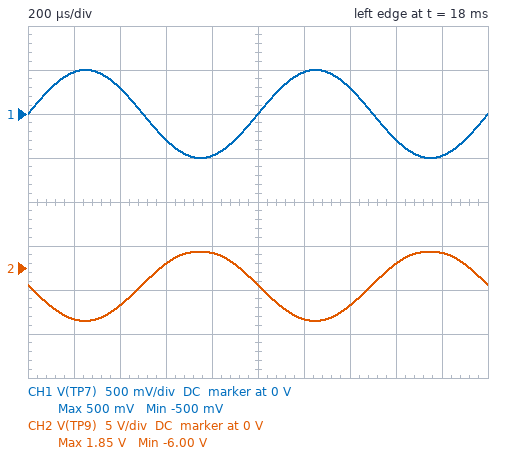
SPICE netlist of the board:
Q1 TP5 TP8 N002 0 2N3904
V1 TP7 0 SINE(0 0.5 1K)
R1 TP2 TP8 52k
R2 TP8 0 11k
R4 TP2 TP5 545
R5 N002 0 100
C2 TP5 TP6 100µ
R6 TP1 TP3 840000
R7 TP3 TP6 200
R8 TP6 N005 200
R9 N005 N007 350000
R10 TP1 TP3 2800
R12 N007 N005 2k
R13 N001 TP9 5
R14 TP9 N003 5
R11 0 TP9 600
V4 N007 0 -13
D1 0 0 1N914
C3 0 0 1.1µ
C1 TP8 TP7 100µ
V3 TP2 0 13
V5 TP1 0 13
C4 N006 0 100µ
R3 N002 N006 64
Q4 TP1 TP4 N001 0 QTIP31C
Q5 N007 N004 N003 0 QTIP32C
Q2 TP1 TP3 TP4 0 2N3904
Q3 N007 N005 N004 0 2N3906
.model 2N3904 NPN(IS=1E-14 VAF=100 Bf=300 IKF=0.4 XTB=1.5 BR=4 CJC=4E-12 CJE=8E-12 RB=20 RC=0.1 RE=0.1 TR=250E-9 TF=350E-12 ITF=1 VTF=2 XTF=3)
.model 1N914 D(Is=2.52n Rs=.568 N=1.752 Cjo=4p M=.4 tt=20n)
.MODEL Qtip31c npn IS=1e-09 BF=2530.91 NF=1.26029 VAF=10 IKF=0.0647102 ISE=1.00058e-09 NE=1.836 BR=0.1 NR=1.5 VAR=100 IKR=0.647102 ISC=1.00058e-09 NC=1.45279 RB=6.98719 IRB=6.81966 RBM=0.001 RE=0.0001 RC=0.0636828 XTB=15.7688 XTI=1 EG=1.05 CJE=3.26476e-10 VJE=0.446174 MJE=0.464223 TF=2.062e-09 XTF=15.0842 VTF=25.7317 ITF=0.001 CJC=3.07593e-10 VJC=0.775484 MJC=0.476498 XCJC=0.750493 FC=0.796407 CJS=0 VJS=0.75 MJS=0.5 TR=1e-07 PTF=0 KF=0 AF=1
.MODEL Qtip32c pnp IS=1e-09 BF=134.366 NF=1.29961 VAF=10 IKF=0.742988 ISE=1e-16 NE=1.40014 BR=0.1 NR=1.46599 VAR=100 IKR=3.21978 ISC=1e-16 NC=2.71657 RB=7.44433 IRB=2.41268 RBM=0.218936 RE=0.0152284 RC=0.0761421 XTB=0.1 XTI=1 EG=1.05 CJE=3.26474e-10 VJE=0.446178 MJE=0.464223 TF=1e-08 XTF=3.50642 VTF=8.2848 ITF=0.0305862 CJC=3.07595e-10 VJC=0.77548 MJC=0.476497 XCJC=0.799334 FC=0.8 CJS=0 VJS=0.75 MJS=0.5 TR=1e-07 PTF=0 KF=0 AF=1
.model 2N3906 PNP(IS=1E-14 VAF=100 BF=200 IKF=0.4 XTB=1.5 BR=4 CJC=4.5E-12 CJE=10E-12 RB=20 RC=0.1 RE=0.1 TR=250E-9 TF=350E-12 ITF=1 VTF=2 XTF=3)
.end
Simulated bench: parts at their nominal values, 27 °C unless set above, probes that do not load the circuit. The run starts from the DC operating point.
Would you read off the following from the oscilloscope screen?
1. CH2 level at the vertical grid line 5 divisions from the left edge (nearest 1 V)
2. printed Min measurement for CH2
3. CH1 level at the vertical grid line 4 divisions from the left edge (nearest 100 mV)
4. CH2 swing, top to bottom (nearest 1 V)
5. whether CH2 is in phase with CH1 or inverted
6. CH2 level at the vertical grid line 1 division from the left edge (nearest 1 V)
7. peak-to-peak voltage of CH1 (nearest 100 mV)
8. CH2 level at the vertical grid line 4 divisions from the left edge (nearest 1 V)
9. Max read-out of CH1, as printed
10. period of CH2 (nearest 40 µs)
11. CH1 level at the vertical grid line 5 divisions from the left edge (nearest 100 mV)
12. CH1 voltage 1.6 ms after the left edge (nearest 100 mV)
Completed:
-2 V
-6.00 V
-500 mV
8 V
inverted
-6 V
1.0 V
2 V
500 mV
1.00 ms
0 V
-300 mV
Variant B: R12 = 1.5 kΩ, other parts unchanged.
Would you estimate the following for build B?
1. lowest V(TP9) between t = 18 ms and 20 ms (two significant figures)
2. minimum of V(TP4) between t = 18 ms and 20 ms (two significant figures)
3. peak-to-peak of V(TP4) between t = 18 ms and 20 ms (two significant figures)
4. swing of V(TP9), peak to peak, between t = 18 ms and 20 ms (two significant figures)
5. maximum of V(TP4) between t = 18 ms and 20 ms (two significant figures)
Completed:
-7.4 V
-7.0 V
7.7 V
7.4 V
680 mV
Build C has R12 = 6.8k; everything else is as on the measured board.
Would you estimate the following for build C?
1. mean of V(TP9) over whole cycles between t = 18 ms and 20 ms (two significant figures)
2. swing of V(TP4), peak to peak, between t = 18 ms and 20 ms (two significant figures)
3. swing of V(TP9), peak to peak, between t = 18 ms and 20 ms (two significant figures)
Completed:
4.6 V
8.9 V
8.7 V
